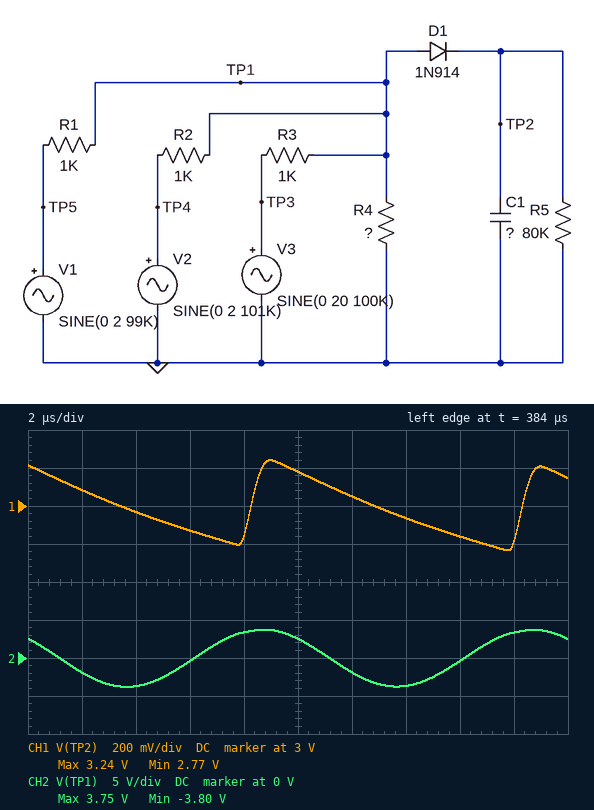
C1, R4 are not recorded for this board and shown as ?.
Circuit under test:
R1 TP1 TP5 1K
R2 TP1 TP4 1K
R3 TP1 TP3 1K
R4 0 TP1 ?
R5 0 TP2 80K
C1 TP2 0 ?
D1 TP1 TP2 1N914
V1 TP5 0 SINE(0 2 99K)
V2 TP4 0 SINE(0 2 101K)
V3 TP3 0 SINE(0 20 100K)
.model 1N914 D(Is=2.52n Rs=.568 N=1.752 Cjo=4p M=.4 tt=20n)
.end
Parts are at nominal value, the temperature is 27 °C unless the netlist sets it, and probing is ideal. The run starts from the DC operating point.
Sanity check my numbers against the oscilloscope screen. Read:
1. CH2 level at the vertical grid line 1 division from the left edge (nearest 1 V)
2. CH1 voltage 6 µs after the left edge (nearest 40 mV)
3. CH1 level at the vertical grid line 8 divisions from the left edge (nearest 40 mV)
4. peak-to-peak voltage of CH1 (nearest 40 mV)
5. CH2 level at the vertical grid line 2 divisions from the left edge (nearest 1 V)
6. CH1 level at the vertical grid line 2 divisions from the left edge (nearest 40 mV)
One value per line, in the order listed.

-2 V
2.88 V
2.84 V
480 mV
-4 V
2.96 V
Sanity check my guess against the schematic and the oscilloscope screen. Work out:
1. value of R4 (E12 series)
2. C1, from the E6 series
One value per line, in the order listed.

680 Ω
680 pF
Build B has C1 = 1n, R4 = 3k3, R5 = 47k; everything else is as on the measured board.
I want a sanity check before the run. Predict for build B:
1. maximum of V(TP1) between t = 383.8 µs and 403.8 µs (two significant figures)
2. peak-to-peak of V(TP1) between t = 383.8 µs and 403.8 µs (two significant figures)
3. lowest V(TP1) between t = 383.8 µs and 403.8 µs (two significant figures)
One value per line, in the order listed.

5.0 V
10 V
-5.1 V
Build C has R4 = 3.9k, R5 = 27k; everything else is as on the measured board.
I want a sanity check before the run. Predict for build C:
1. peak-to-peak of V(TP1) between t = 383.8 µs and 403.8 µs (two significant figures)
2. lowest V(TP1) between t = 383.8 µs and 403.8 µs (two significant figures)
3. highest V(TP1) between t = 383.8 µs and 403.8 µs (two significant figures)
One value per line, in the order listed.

10 V
-5.2 V
5.1 V
